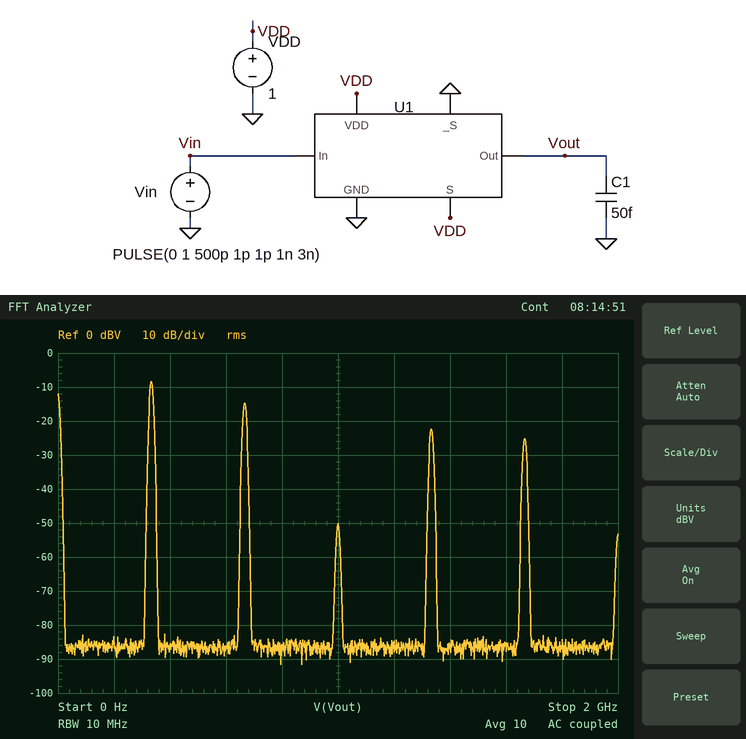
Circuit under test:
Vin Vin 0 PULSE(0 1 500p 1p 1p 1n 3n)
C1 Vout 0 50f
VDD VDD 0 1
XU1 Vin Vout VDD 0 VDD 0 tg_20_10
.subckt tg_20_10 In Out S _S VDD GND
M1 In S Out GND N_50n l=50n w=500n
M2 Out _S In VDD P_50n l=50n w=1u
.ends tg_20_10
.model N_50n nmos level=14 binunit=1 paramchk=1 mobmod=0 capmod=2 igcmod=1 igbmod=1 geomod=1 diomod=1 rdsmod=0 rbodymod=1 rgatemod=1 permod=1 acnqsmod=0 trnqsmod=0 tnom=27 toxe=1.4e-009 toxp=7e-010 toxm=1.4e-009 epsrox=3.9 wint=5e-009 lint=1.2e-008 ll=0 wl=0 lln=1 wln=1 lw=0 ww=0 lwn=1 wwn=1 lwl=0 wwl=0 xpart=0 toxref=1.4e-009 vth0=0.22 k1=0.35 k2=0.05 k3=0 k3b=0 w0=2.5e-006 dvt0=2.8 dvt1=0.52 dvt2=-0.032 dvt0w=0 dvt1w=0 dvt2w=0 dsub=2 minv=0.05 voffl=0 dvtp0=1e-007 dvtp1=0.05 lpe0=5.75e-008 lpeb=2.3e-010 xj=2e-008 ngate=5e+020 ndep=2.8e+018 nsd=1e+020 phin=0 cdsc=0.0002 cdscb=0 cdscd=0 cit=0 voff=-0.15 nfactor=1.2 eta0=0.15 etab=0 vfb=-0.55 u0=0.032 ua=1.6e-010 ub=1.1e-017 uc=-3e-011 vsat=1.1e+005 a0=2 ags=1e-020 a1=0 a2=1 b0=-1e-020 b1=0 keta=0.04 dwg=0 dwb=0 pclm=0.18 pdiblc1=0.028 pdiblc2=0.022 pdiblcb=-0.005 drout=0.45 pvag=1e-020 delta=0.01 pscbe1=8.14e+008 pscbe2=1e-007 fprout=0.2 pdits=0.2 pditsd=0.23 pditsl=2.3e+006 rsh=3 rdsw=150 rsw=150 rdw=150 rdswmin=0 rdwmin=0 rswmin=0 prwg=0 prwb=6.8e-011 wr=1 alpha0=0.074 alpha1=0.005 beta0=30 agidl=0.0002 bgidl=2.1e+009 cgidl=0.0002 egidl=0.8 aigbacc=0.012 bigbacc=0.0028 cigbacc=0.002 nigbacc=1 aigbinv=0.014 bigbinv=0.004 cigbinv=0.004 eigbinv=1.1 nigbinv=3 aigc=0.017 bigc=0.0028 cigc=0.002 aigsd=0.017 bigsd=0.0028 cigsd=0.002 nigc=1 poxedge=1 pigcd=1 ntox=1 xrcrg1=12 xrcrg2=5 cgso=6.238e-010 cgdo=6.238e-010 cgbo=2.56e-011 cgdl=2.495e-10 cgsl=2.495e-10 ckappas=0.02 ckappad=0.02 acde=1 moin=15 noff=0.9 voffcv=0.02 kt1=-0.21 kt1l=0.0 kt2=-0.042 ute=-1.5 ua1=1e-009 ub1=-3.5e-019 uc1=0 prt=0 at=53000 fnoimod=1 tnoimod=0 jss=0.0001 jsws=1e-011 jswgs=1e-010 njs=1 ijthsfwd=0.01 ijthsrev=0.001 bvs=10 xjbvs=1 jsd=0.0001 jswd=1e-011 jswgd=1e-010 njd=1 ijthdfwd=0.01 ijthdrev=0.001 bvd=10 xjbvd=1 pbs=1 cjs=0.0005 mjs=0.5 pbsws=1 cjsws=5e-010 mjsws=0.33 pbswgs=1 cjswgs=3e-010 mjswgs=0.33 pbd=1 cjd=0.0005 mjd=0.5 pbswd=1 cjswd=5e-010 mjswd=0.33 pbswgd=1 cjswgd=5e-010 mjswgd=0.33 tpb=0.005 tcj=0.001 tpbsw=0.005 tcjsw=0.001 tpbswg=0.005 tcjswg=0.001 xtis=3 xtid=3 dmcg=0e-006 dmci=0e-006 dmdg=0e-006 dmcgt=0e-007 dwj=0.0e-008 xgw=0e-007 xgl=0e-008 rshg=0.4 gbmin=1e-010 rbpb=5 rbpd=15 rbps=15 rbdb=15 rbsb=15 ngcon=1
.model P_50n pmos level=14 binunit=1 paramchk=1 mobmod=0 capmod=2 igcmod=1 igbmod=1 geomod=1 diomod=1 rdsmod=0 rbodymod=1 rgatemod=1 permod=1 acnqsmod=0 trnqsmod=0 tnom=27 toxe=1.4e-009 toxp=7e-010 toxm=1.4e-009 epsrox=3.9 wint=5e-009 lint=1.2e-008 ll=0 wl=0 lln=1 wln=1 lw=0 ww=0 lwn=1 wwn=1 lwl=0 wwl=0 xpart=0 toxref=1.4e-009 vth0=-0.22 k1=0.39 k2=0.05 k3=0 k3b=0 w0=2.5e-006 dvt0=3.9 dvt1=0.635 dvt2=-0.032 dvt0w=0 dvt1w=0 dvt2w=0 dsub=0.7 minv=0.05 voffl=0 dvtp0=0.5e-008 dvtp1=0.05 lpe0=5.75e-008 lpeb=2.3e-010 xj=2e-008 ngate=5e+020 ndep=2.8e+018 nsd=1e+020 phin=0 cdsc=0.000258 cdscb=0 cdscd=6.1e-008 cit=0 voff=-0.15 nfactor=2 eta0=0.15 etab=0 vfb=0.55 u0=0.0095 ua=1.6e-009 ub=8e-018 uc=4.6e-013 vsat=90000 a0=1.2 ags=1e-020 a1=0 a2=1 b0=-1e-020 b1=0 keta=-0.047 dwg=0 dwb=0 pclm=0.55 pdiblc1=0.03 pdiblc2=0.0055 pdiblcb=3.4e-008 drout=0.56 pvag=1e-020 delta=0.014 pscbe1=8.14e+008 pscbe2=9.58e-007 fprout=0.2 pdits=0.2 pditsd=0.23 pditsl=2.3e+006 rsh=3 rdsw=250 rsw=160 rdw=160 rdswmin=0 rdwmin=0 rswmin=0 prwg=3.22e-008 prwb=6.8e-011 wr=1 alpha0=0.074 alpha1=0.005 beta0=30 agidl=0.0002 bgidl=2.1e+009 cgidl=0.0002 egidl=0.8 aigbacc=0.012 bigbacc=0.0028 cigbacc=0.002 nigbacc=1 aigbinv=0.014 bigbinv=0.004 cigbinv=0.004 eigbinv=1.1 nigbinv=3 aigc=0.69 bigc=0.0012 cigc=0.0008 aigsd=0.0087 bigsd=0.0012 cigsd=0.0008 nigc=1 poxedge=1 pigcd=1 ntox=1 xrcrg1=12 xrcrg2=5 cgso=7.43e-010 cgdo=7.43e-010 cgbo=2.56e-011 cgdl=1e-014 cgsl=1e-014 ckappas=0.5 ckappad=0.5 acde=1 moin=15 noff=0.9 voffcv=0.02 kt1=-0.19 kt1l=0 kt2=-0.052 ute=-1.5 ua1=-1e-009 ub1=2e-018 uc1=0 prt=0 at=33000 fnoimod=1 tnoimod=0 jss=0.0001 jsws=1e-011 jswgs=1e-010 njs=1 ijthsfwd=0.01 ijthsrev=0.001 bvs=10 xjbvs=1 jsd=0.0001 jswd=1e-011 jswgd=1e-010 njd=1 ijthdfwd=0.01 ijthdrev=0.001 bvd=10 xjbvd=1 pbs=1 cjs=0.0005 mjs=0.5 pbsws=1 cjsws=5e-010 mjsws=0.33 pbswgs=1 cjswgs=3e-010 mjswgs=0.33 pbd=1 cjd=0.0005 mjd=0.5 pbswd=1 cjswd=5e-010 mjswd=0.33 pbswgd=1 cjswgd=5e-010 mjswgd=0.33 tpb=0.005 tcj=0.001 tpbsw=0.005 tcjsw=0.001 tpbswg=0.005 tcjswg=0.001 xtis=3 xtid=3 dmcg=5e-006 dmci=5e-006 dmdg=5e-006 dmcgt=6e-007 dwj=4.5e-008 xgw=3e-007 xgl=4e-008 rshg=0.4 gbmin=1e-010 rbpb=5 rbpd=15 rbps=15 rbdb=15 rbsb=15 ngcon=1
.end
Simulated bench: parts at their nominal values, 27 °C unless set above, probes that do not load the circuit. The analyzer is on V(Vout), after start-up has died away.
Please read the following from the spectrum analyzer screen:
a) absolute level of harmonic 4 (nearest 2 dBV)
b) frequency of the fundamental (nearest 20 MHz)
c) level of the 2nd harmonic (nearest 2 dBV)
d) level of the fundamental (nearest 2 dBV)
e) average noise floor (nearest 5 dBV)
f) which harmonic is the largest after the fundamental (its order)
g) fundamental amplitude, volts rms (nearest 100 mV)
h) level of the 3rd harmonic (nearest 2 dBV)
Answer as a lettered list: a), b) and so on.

a) -22 dBV
b) 340 MHz
c) -14 dBV
d) -8 dBV
e) -85 dBV
f) 2
g) 400 mV
h) -50 dBV
